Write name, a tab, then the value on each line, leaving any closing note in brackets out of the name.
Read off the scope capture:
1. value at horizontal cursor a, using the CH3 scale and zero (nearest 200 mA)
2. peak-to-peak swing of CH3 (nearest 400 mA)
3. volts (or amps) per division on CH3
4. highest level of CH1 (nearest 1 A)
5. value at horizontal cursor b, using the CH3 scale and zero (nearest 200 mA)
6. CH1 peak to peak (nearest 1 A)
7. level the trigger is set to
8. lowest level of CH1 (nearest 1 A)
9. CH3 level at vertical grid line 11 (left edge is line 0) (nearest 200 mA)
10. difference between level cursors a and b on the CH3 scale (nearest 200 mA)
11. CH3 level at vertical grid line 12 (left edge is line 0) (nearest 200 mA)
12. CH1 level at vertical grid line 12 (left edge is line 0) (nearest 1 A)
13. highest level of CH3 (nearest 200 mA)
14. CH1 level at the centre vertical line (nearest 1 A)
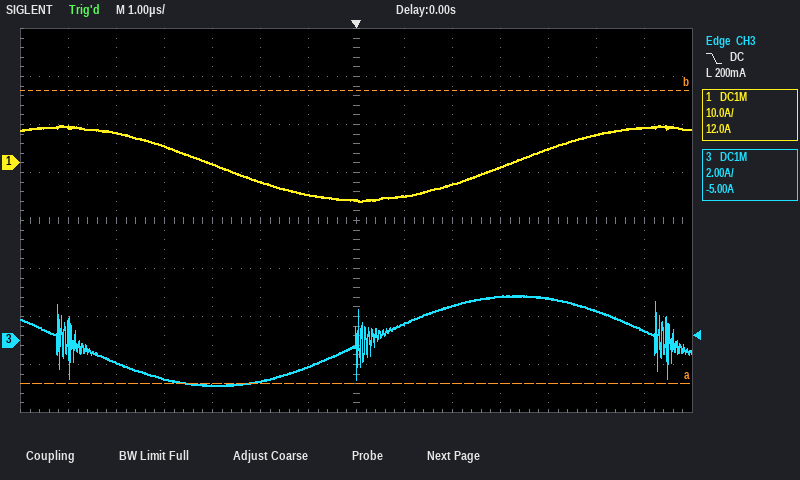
value at horizontal cursor a, using the CH3 scale and zero	-1.8 A
peak-to-peak swing of CH3	3.6 A
volts (or amps) per division on CH3	2 A
highest level of CH1	8 A
value at horizontal cursor b, using the CH3 scale and zero	10.4 A
CH1 peak to peak	16 A
level the trigger is set to	200 mA
lowest level of CH1	-8 A
CH3 level at vertical grid line 11 (left edge is line 0)	1.8 A
difference between level cursors a and b on the CH3 scale	12.2 A
CH3 level at vertical grid line 12 (left edge is line 0)	1.2 A
CH1 level at vertical grid line 12 (left edge is line 0)	6 A
highest level of CH3	1.8 A
CH1 level at the centre vertical line	-8 A
